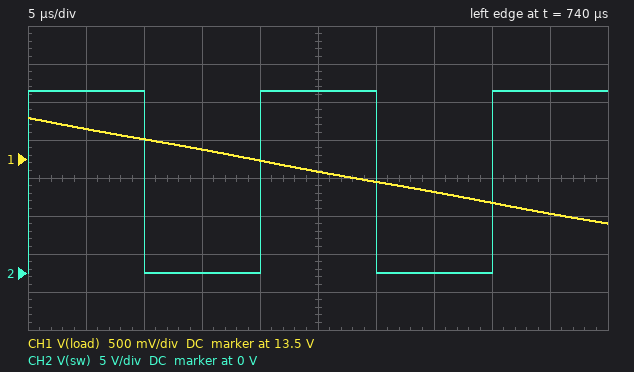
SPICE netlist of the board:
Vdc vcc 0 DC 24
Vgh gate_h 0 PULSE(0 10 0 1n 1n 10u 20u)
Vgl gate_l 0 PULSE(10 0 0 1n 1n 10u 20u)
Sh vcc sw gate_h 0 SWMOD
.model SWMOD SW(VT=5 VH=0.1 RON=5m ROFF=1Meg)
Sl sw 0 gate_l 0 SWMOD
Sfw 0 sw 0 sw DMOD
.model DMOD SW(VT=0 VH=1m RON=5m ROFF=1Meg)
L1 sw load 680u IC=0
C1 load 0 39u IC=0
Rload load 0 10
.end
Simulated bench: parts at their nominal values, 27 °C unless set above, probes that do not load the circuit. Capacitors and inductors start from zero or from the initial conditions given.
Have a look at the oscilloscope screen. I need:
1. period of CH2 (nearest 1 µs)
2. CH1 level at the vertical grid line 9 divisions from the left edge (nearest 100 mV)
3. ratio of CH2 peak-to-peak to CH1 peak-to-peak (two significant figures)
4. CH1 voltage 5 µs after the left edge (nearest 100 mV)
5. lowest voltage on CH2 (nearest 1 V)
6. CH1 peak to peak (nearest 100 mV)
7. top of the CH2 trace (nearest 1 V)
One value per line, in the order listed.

20 µs
12.8 V
17
13.9 V
0 V
1.4 V
24 V
